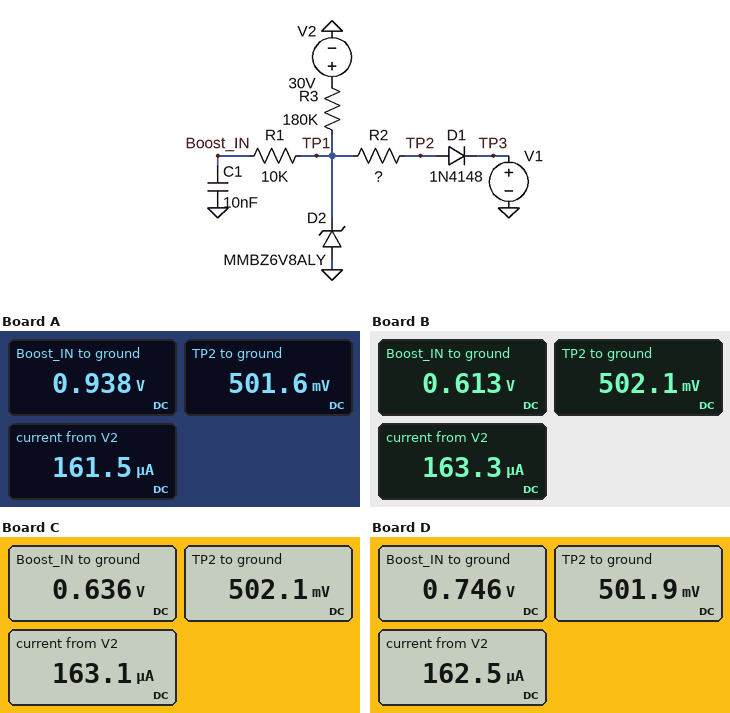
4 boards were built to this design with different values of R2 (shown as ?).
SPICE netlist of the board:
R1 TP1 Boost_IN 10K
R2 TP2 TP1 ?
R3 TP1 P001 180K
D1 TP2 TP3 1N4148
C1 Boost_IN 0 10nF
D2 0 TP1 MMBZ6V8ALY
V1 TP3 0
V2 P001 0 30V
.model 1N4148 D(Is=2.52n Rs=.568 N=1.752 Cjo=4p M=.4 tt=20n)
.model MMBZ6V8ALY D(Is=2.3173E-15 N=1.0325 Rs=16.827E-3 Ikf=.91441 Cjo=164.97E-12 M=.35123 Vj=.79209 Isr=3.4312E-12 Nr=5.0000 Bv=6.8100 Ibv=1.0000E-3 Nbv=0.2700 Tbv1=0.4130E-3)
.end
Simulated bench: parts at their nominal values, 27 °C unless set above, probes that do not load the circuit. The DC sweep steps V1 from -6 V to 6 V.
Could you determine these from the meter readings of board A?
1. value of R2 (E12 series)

2.7 kΩ
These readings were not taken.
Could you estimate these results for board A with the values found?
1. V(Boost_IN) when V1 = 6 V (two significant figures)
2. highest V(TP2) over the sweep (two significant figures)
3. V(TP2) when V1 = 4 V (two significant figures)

6.8 V
6.5 V
4.5 V
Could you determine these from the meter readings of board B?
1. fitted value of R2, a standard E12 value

680 Ω
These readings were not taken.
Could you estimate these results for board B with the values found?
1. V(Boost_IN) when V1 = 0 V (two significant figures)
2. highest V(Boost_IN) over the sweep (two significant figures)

610 mV
6.6 V
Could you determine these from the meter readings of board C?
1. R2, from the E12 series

820 Ω
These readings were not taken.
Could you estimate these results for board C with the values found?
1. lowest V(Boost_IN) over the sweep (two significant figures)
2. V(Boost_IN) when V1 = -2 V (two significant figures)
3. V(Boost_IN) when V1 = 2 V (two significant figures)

-760 mV
-710 mV
2.6 V
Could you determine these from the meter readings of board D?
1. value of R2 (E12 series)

1.5 kΩ
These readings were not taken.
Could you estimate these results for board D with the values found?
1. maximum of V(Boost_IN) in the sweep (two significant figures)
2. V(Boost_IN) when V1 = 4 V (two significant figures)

6.7 V
4.7 V
